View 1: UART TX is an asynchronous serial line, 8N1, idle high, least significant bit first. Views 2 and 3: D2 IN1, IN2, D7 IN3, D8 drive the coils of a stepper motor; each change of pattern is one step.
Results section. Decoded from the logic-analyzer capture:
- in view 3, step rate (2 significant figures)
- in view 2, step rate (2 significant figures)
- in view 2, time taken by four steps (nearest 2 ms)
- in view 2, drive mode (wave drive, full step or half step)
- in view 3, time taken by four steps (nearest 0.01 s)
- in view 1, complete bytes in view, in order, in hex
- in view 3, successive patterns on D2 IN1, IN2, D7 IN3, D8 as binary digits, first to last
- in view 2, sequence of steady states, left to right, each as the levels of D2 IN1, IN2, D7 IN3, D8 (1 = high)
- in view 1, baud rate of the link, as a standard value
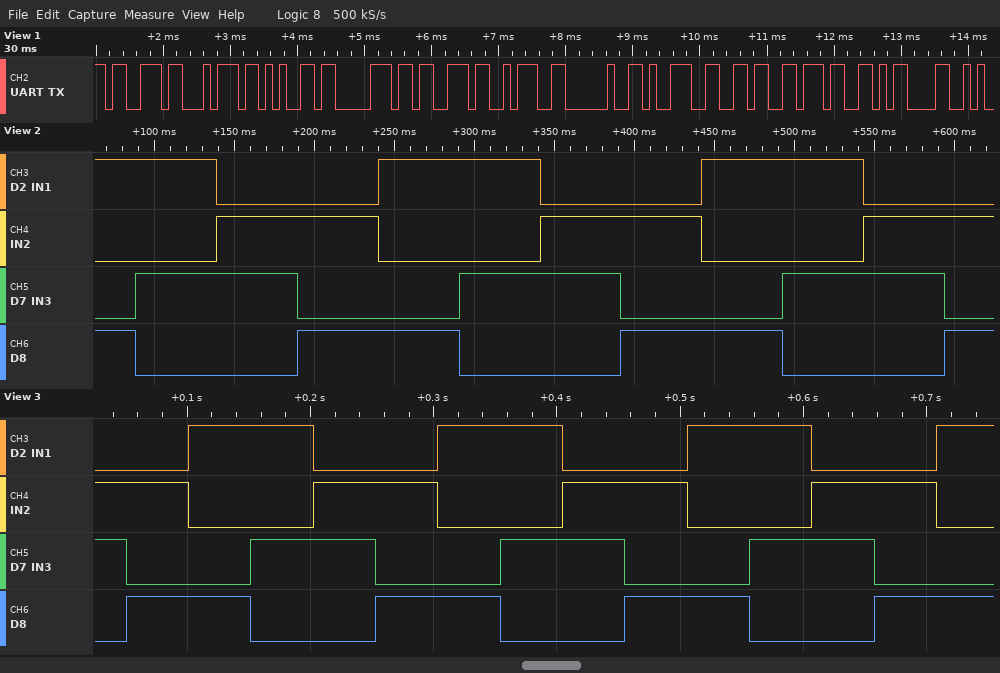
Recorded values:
20 steps/s
20 steps/s
202 ms
full step
0.20 s
73 74 65 70 73 3A 20 39 36 37 0D
0110 0101 1001 1010 0110 0101 1001 1010 0110 0101 1001 1010 0110 0101 1001
1001 1010 0110 0101 1001 1010 0110 0101 1001 1010 0110 0101
9600 baud
